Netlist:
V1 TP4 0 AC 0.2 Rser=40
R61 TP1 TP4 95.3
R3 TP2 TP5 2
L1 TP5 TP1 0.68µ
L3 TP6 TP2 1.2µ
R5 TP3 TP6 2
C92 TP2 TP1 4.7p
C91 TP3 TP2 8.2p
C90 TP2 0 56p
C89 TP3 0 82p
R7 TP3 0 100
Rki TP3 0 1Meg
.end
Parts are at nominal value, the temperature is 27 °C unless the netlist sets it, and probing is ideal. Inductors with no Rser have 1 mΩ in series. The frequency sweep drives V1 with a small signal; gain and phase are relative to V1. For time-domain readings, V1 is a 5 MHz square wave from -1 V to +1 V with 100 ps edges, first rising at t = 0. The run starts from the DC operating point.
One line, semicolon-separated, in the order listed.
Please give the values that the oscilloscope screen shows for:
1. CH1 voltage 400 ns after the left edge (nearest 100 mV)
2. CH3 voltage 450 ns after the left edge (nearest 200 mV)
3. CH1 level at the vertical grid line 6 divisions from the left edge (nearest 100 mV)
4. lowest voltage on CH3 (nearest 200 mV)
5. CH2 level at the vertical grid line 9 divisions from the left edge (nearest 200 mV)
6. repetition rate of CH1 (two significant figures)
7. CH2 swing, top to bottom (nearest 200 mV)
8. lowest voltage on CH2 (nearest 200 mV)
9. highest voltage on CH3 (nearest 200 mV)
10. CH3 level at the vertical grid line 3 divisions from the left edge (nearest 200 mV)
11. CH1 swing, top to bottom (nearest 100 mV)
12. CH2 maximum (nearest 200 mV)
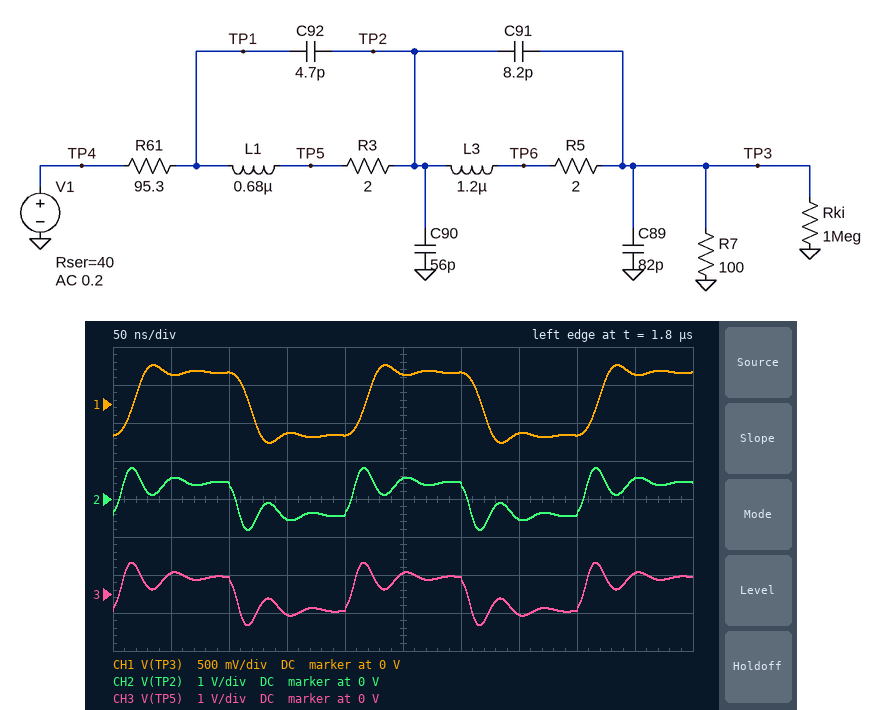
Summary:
-400 mV; 600 mV; 400 mV; -800 mV; 600 mV; 5.0 MHz; 1.6 V; -800 mV; 800 mV; -600 mV; 1.0 V; 800 mV
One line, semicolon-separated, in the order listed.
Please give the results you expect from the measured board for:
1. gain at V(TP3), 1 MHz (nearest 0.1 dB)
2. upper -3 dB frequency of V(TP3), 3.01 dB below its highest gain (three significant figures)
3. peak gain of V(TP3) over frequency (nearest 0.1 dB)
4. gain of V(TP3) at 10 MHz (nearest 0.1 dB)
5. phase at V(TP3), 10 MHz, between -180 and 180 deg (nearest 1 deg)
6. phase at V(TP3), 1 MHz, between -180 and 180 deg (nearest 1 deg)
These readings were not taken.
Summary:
-7.6 dB; 25.9 MHz; -7.6 dB; -7.9 dB; -59 deg; -6 deg
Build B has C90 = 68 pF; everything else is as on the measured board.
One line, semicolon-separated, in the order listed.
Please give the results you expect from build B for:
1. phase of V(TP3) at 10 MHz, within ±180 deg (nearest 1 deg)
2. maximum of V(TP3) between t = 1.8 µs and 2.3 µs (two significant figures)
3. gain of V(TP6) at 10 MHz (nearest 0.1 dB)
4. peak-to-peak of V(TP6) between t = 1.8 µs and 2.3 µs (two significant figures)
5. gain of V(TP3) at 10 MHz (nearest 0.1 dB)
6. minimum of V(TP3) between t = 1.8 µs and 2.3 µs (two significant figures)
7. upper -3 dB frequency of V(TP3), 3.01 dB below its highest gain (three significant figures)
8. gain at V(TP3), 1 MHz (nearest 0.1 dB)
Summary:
-61 deg; 520 mV; -7.6 dB; 1.1 V; -7.8 dB; -520 mV; 24.9 MHz; -7.6 dB
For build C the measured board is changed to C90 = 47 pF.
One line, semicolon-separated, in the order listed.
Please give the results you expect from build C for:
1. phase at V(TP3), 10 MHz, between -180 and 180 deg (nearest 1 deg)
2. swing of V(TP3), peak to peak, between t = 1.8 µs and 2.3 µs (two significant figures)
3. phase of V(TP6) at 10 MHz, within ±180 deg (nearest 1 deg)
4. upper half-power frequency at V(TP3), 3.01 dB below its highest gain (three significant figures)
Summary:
-57 deg; 990 mV; -56 deg; 26.3 MHz
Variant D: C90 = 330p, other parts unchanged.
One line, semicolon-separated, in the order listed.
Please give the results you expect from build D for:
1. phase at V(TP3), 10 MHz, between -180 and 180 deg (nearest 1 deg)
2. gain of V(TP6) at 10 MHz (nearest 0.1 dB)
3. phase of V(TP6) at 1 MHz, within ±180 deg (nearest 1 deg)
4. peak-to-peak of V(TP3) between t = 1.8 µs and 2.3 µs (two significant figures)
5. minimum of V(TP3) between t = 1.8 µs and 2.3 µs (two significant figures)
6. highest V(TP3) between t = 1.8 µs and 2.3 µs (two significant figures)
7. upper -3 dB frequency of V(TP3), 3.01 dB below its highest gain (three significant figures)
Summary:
-109 deg; -9.8 dB; -11 deg; 840 mV; -420 mV; 420 mV; 11.4 MHz
